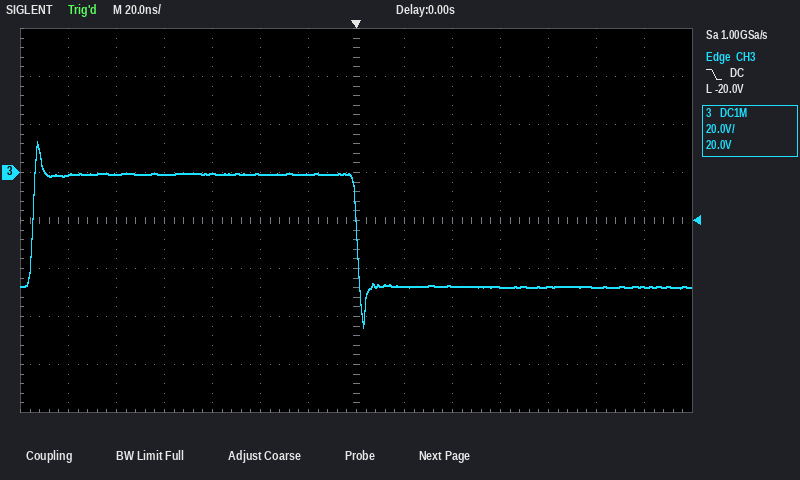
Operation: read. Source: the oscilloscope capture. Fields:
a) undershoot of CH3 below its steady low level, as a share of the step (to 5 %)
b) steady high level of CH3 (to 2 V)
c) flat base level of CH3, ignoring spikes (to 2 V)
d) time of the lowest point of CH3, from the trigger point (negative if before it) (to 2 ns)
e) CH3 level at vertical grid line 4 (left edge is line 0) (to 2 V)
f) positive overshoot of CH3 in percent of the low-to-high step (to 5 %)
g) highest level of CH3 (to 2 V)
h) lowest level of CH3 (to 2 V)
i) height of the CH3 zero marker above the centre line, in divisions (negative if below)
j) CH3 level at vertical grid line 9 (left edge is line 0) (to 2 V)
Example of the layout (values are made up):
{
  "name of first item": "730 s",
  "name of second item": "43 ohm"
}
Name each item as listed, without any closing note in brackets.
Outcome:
{
  "undershoot of CH3 below its steady low level, as a share of the step": "35 %",
  "steady high level of CH3": "0 V",
  "flat base level of CH3, ignoring spikes": "-48 V",
  "time of the lowest point of CH3, from the trigger point (negative if before it)": "+4 ns",
  "CH3 level at vertical grid line 4 (left edge is line 0)": "0 V",
  "positive overshoot of CH3 in percent of the low-to-high step": "30 %",
  "highest level of CH3": "12 V",
  "lowest level of CH3": "-64 V",
  "height of the CH3 zero marker above the centre line, in divisions": "+1.0 div",
  "CH3 level at vertical grid line 9 (left edge is line 0)": "-48 V"
}
